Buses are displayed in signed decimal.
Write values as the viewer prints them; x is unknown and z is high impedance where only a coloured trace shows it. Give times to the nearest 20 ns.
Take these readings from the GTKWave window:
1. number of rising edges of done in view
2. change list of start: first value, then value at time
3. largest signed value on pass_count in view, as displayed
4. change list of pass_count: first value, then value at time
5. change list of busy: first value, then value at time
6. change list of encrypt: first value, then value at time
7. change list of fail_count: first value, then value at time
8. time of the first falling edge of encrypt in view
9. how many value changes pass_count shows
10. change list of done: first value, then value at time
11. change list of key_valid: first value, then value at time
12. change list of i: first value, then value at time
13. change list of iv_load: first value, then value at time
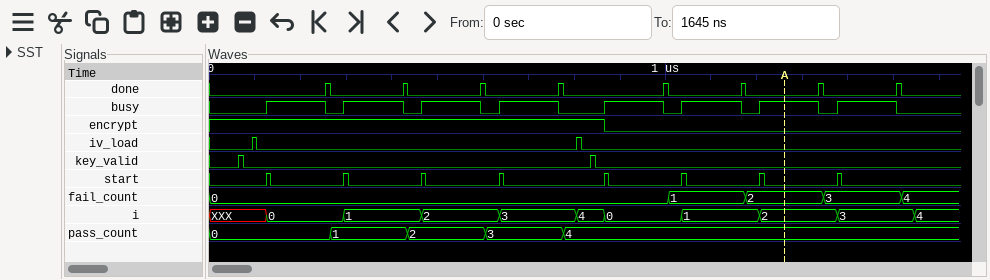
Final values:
8
0, 1 at 120 ns, 0 at 140 ns, 1 at 300 ns, 0 at 300 ns, 1 at 460 ns, 0 at 480 ns, 1 at 640 ns, 0 at 640 ns, 1 at 860 ns, 0 at 880 ns, 1 at 1040 ns, 0 at 1040 ns, 1 at 1200 ns, 0 at 1220 ns, 1 at 1380 ns, 0 at 1380 ns
4
0, 1 at 260 ns, 2 at 440 ns, 3 at 600 ns, 4 at 780 ns
0, 1 at 120 ns, 0 at 260 ns, 1 at 300 ns, 0 at 420 ns, 1 at 460 ns, 0 at 600 ns, 1 at 640 ns, 0 at 760 ns, 1 at 860 ns, 0 at 1000 ns, 1 at 1040 ns, 0 at 1160 ns, 1 at 1200 ns, 0 at 1340 ns, 1 at 1380 ns, 0 at 1500 ns
1, 0 at 860 ns
0, 1 at 1000 ns, 2 at 1180 ns, 3 at 1340 ns, 4 at 1520 ns
860 ns
4
0, 1 at 260 ns, 0 at 260 ns, 1 at 420 ns, 0 at 440 ns, 1 at 600 ns, 0 at 600 ns, 1 at 760 ns, 0 at 780 ns, 1 at 1000 ns, 0 at 1000 ns, 1 at 1160 ns, 0 at 1180 ns, 1 at 1340 ns, 0 at 1340 ns, 1 at 1500 ns, 0 at 1520 ns
0, 1 at 60 ns, 0 at 80 ns, 1 at 840 ns, 0 at 840 ns
XXX, 0 at 120 ns, 1 at 300 ns, 2 at 460 ns, 3 at 640 ns, 4 at 800 ns, 0 at 860 ns, 1 at 1040 ns, 2 at 1200 ns, 3 at 1380 ns, 4 at 1540 ns
0, 1 at 100 ns, 0 at 100 ns, 1 at 800 ns, 0 at 820 ns
